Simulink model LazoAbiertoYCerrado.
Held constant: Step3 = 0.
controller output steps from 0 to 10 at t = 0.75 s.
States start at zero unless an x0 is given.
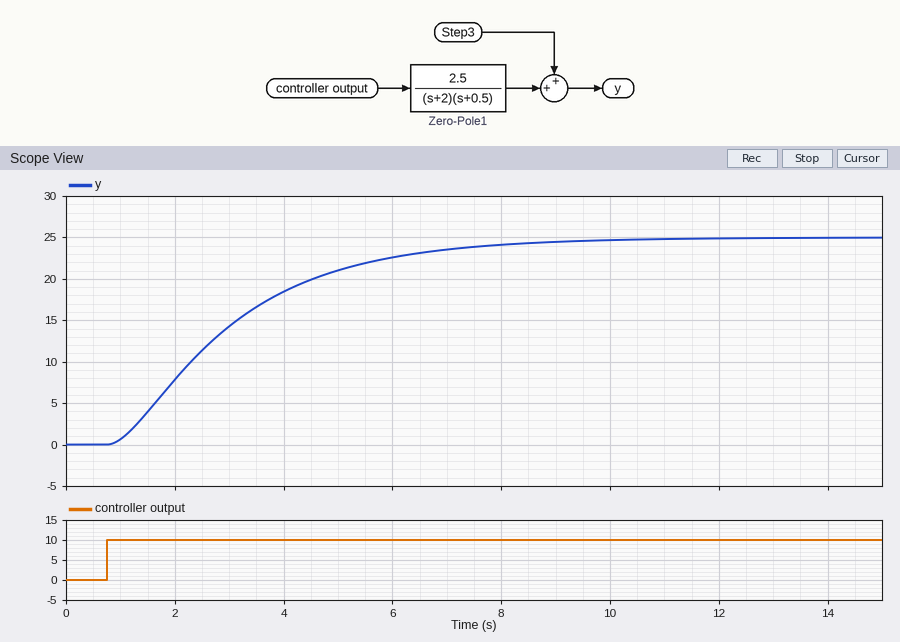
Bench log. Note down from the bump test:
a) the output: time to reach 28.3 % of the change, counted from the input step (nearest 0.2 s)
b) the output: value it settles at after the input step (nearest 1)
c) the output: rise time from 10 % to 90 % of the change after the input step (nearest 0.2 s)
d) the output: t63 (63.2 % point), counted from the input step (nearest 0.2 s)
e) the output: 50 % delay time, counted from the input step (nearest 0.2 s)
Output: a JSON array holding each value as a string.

["1.2 s", "25", "4.6 s", "2.6 s", "2.0 s"]
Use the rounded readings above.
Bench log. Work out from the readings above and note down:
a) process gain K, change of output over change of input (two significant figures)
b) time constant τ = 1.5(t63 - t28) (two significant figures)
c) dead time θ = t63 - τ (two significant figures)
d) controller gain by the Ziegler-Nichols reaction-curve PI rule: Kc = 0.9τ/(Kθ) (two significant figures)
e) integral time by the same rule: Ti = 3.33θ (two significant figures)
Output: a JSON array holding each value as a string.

["2.5", "2.1 s", "0.50 s", "1.5", "1.7 s"]
